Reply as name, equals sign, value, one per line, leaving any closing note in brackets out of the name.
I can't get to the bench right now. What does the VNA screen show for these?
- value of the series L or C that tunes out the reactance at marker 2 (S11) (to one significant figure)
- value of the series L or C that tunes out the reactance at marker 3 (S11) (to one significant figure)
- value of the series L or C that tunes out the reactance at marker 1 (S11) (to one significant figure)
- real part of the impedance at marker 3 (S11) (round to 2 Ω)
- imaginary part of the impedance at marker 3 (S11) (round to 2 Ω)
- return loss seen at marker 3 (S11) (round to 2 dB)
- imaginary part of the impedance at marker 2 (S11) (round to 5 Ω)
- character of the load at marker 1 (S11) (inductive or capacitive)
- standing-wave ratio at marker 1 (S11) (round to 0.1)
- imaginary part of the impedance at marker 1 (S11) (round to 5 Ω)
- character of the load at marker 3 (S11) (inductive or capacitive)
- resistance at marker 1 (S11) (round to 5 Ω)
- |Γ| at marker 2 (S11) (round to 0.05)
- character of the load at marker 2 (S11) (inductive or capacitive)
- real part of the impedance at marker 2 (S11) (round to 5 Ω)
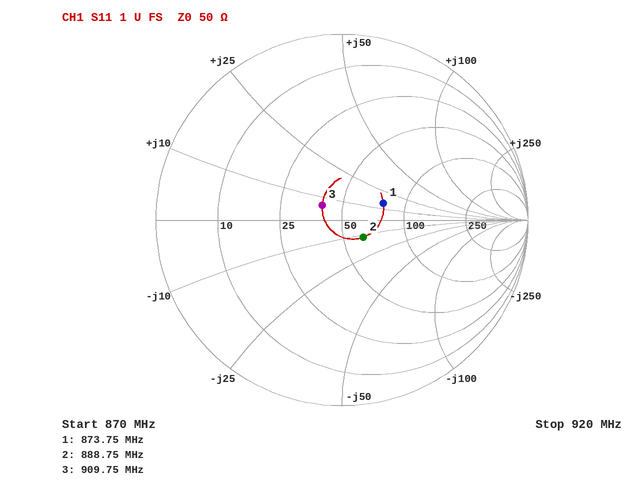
value of the series L or C that tunes out the reactance at marker 2 (S11) = 2 nH
value of the series L or C that tunes out the reactance at marker 3 (S11) = 30 pF
value of the series L or C that tunes out the reactance at marker 1 (S11) = 10 pF
real part of the impedance at marker 3 (S11) = 40 Ω
imaginary part of the impedance at marker 3 (S11) = +6 Ω
return loss seen at marker 3 (S11) = 18 dB
imaginary part of the impedance at marker 2 (S11) = -10 Ω
character of the load at marker 1 (S11) = inductive
standing-wave ratio at marker 1 (S11) = 1.6
imaginary part of the impedance at marker 1 (S11) = +15 Ω
character of the load at marker 3 (S11) = inductive
resistance at marker 1 (S11) = 75 Ω
|Γ| at marker 2 (S11) = 0.15
character of the load at marker 2 (S11) = capacitive
real part of the impedance at marker 2 (S11) = 60 Ω
